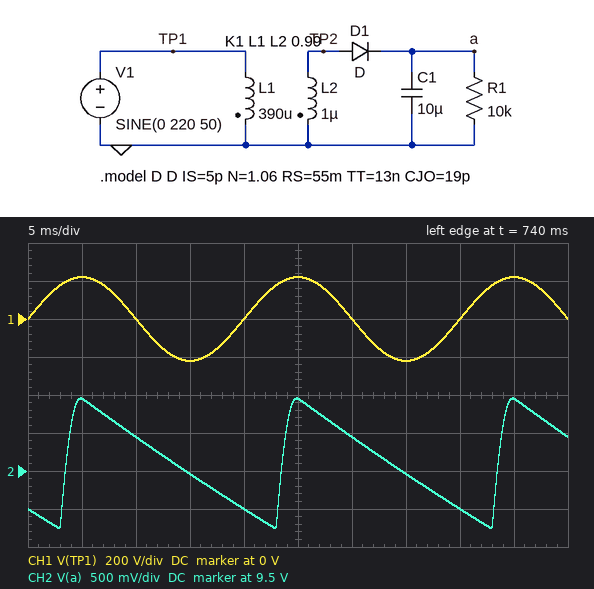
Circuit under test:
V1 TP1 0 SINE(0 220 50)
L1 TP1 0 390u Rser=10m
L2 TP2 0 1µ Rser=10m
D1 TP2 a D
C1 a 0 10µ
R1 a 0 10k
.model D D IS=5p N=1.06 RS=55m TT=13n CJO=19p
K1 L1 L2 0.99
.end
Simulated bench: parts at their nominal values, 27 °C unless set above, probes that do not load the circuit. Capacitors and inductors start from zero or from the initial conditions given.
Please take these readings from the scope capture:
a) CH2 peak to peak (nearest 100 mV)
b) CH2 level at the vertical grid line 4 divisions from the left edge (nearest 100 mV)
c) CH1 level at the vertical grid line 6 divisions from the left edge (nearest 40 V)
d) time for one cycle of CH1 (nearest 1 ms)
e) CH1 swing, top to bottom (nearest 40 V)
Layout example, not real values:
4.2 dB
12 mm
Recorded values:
1.7 V
9.0 V
0 V
20 ms
440 V
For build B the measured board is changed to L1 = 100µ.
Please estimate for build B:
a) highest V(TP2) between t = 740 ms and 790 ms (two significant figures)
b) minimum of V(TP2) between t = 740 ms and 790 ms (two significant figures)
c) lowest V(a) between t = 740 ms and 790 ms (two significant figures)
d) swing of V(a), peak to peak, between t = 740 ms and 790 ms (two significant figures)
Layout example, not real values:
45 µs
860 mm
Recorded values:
21 V
-21 V
17 V
3.3 V
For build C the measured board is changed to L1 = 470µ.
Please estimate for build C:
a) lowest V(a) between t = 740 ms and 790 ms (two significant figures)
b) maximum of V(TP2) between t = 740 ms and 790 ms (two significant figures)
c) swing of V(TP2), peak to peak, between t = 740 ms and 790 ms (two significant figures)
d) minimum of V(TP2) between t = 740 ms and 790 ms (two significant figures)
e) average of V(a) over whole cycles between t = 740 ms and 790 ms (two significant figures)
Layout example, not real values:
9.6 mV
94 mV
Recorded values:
7.9 V
10 V
20 V
-10 V
8.7 V
